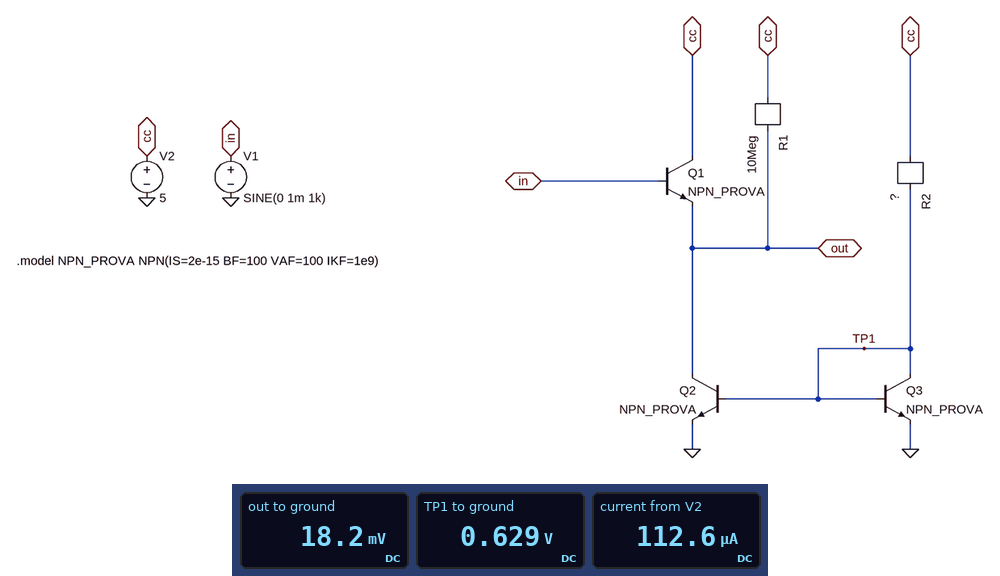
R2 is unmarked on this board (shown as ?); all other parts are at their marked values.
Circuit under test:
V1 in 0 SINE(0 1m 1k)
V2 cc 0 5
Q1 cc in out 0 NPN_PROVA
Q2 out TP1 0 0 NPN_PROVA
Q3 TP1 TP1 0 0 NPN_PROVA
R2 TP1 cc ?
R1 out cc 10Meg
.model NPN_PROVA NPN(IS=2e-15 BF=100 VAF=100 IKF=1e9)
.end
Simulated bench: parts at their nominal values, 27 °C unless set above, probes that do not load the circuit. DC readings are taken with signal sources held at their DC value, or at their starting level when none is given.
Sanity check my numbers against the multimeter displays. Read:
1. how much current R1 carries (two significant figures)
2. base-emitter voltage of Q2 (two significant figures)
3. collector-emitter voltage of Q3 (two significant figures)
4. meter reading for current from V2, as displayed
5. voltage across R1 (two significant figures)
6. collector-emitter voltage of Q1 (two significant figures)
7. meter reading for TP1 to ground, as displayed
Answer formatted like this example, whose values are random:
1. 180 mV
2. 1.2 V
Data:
1. 500 nA
2. 630 mV
3. 630 mV
4. 112.6 µA
5. 5.0 V
6. 5.0 V
7. 0.629 V
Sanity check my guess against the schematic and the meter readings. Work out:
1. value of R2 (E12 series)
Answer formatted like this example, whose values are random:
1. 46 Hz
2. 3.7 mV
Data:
1. 39 kΩ
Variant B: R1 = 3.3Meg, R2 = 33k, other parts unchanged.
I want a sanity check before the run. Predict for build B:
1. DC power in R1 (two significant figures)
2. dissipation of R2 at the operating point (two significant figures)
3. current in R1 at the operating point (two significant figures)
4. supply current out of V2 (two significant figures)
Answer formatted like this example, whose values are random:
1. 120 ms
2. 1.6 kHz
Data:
1. 7.5 µW
2. 580 µW
3. 1.5 µA
4. 130 µA
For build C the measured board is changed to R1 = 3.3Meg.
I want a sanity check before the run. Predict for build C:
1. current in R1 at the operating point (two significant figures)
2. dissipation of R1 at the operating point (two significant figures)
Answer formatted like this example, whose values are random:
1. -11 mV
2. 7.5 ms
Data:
1. 1.5 µA
2. 7.5 µW
